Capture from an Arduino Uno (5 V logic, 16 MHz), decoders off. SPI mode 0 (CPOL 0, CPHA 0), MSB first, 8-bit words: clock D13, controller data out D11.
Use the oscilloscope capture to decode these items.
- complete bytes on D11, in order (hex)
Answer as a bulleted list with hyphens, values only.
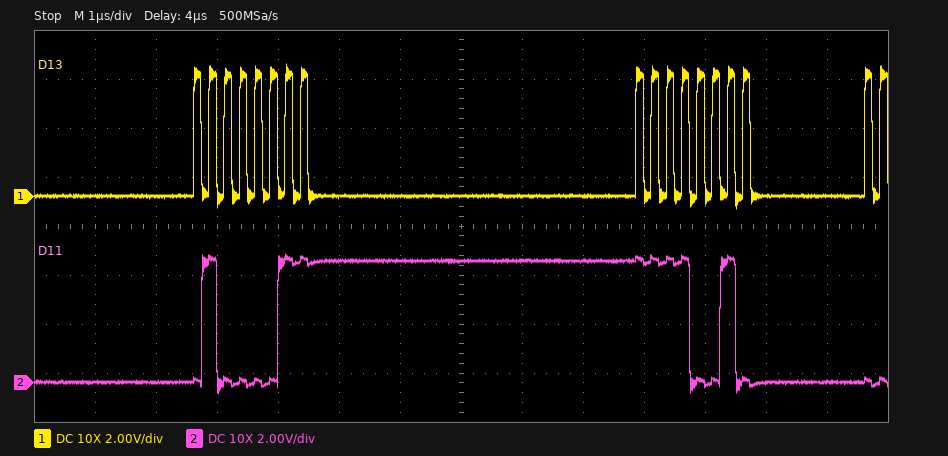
- 0x43 0xF2
